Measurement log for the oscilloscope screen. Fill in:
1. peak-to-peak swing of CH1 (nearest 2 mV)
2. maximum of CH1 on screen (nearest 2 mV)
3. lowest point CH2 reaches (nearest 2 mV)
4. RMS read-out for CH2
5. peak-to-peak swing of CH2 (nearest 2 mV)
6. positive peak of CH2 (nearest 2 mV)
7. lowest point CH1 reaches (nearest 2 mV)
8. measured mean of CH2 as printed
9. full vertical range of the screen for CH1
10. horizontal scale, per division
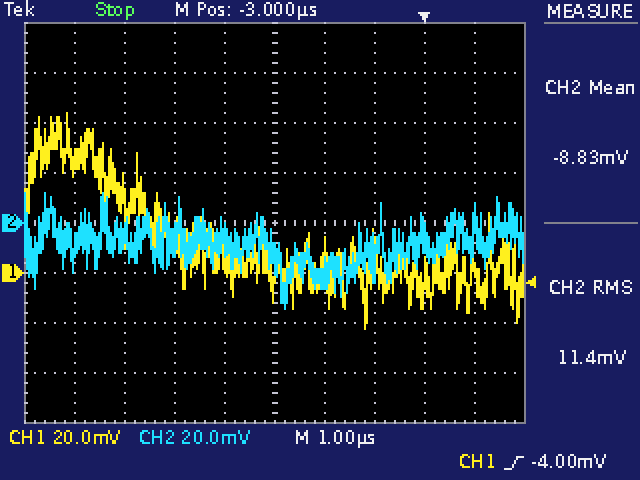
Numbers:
86 mV
64 mV
-34 mV
11.4 mV
46 mV
12 mV
-22 mV
-8.83 mV
160 mV
1 µs
